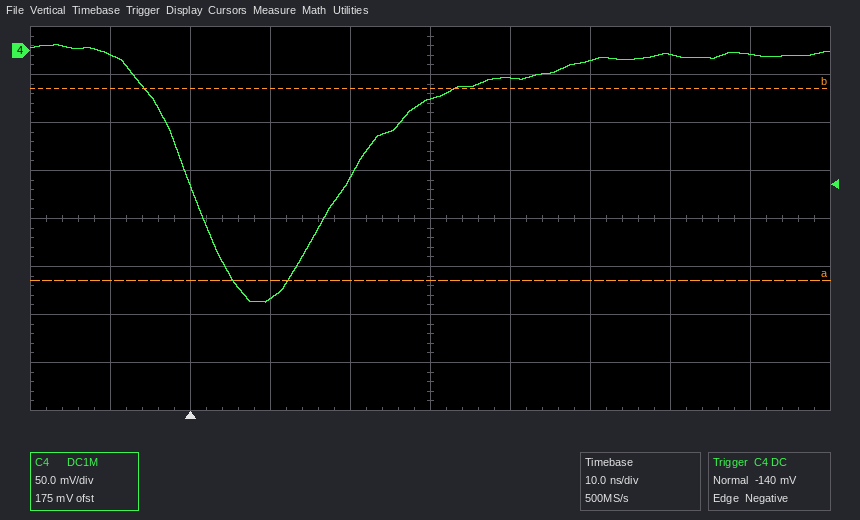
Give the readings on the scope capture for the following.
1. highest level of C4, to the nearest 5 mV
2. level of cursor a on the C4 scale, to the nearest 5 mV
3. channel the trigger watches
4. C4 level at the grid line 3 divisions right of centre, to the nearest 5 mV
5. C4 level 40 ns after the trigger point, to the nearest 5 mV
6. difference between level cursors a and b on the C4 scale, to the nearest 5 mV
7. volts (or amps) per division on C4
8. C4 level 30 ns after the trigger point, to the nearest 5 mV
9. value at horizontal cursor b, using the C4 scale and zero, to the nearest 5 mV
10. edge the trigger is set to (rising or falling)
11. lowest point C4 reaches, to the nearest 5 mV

5 mV
-240 mV
C4
-5 mV
-30 mV
200 mV
50 mV
-50 mV
-40 mV
falling
-260 mV
